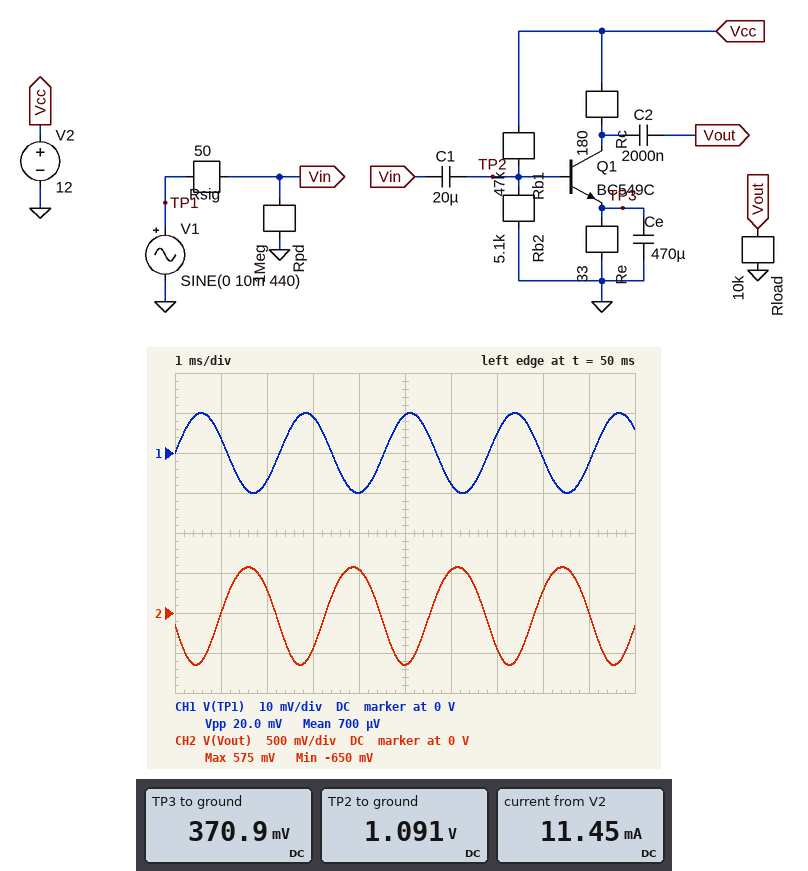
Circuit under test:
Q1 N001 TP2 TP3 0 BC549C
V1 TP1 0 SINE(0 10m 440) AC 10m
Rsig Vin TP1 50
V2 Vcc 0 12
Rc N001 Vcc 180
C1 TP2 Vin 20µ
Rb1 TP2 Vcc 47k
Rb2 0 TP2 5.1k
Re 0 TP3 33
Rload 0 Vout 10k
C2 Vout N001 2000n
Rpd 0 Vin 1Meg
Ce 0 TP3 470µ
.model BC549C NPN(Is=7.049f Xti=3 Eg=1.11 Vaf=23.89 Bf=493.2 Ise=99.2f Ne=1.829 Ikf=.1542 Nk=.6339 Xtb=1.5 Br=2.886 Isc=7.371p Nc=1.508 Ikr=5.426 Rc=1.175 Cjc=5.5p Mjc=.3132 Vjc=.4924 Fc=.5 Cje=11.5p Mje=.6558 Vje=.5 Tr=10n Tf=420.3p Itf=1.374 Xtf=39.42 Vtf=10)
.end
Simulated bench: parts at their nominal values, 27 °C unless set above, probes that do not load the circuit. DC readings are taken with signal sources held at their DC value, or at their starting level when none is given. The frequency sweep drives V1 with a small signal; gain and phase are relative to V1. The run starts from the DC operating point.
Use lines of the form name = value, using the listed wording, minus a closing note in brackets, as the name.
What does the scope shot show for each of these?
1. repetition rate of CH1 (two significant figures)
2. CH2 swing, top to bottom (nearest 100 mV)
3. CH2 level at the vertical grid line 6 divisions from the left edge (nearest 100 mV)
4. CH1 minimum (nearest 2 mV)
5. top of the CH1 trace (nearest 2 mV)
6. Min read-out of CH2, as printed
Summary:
repetition rate of CH1 = 440 Hz
CH2 swing, top to bottom = 1.2 V
CH2 level at the vertical grid line 6 divisions from the left edge = 500 mV
CH1 minimum = -10 mV
top of the CH1 trace = 10 mV
Min read-out of CH2, as printed = -650 mV
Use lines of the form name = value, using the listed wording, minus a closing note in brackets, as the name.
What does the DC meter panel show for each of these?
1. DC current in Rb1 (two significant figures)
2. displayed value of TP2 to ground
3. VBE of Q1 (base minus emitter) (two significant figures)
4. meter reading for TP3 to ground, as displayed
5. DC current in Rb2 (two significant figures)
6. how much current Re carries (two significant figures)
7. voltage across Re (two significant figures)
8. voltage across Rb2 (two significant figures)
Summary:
DC current in Rb1 = 230 µA
displayed value of TP2 to ground = 1.091 V
VBE of Q1 (base minus emitter) = 720 mV
meter reading for TP3 to ground, as displayed = 370.9 mV
DC current in Rb2 = 210 µA
how much current Re carries = 11 mA
voltage across Re = 370 mV
voltage across Rb2 = 1.1 V
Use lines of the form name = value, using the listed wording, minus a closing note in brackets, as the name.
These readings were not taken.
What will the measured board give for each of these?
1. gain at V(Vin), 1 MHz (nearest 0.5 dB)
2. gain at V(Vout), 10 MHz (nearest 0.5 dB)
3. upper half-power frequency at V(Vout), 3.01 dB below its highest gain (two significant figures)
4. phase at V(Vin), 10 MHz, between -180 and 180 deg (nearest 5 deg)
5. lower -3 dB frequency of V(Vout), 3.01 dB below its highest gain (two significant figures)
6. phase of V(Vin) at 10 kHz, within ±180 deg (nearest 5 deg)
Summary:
gain at V(Vin), 1 MHz = -0.5 dB
gain at V(Vout), 10 MHz = 33.0 dB
upper half-power frequency at V(Vout), 3.01 dB below its highest gain = 9.3 MHz
phase at V(Vin), 10 MHz, between -180 and 180 deg = -45 deg
lower -3 dB frequency of V(Vout), 3.01 dB below its highest gain = 140 Hz
phase of V(Vin) at 10 kHz, within ±180 deg = 0 deg
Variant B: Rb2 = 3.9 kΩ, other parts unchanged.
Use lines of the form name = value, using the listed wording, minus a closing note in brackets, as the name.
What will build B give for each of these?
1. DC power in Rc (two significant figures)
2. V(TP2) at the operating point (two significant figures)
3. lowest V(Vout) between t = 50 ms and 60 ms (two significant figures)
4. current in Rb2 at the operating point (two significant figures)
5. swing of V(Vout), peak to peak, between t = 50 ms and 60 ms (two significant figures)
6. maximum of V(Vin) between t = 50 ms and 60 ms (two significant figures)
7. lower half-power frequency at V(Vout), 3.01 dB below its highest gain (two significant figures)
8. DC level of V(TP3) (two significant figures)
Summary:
DC power in Rc = 5.8 mW
V(TP2) at the operating point = 890 mV
lowest V(Vout) between t = 50 ms and 60 ms = -370 mV
current in Rb2 at the operating point = 230 µA
swing of V(Vout), peak to peak, between t = 50 ms and 60 ms = 690 mV
maximum of V(Vin) between t = 50 ms and 60 ms = 9.7 mV
lower half-power frequency at V(Vout), 3.01 dB below its highest gain = 81 Hz
DC level of V(TP3) = 190 mV
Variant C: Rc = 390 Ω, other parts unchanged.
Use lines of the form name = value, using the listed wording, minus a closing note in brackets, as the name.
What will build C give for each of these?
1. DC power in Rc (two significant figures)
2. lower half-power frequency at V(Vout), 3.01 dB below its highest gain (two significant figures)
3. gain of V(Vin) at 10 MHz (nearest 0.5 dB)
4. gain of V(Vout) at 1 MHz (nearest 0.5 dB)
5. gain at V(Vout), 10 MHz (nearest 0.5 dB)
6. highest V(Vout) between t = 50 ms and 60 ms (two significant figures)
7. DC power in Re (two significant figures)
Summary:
DC power in Rc = 47 mW
lower half-power frequency at V(Vout), 3.01 dB below its highest gain = 130 Hz
gain of V(Vin) at 10 MHz = -5.5 dB
gain of V(Vout) at 1 MHz = 42.0 dB
gain at V(Vout), 10 MHz = 36.5 dB
highest V(Vout) between t = 50 ms and 60 ms = 1.1 V
DC power in Re = 4.0 mW
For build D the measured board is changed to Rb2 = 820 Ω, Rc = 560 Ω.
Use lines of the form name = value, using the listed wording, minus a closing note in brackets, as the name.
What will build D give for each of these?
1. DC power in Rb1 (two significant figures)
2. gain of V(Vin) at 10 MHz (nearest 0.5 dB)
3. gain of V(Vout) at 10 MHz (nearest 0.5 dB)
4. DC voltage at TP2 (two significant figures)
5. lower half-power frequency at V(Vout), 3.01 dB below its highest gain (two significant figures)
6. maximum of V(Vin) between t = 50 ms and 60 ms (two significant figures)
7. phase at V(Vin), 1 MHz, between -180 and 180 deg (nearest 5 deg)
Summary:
DC power in Rb1 = 3.0 mW
gain of V(Vin) at 10 MHz = -0.5 dB
gain of V(Vout) at 10 MHz = -24.0 dB
DC voltage at TP2 = 210 mV
lower half-power frequency at V(Vout), 3.01 dB below its highest gain = 70 MHz
maximum of V(Vin) between t = 50 ms and 60 ms = 9.4 mV
phase at V(Vin), 1 MHz, between -180 and 180 deg = 0 deg
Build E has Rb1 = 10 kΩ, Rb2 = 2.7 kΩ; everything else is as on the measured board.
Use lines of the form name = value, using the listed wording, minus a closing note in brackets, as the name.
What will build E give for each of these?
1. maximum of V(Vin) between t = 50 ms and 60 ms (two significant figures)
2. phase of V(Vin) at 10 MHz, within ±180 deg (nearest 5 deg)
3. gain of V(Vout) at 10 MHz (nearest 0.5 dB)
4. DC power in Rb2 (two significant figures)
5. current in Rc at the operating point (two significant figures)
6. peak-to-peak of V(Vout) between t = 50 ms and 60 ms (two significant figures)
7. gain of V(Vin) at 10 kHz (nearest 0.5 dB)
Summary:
maximum of V(Vin) between t = 50 ms and 60 ms = 8.6 mV
phase of V(Vin) at 10 MHz, within ±180 deg = -70 deg
gain of V(Vout) at 10 MHz = 32.5 dB
DC power in Rb2 = 1.9 mW
current in Rc at the operating point = 46 mA
peak-to-peak of V(Vout) between t = 50 ms and 60 ms = 2.3 V
gain of V(Vin) at 10 kHz = -2.0 dB
